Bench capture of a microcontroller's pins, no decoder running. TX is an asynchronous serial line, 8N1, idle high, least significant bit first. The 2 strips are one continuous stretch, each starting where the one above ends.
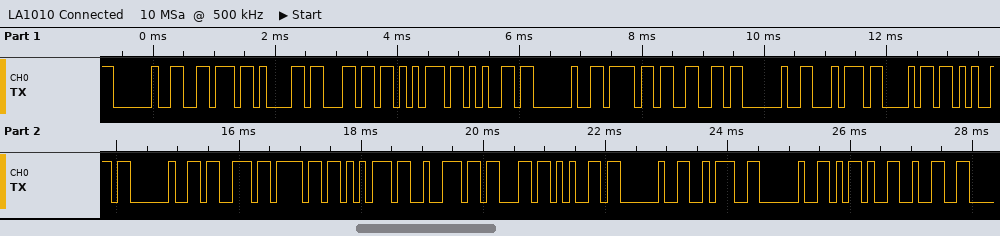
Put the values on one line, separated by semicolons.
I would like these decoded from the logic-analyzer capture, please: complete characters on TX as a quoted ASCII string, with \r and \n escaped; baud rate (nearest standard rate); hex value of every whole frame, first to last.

" value of the source : -2"; 9600 baud; 20 76 61 6C 75 65 20 6F 66 20 74 68 65 20 73 6F 75 72 63 65 20 3A 20 2D 32
